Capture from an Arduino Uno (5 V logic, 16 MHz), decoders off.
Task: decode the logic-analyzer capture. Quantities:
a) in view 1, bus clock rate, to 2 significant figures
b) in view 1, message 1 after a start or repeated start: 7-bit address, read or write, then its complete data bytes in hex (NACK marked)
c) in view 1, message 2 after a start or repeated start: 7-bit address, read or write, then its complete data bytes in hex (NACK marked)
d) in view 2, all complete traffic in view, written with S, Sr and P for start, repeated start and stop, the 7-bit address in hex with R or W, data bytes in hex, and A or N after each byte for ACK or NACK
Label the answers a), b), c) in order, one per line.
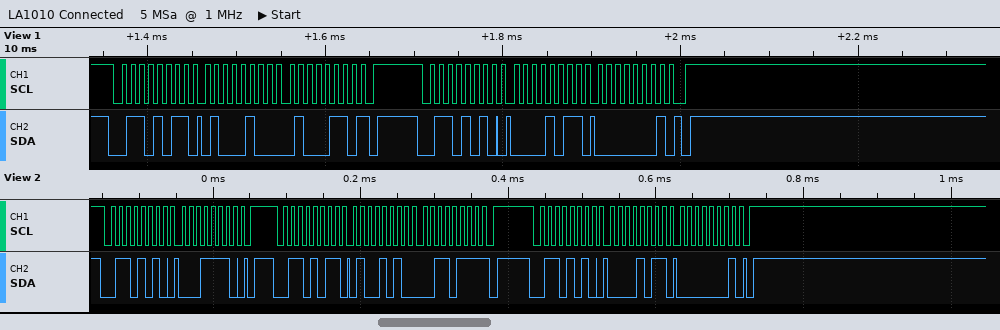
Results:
a) 100 kHz
b) 0x35 read: 44 46 NACK
c) 0x35 write: 0B 01
d) S 35W A 1E A P S 35R A 4A A 37 N P S 35W A 0B A 01 A P
